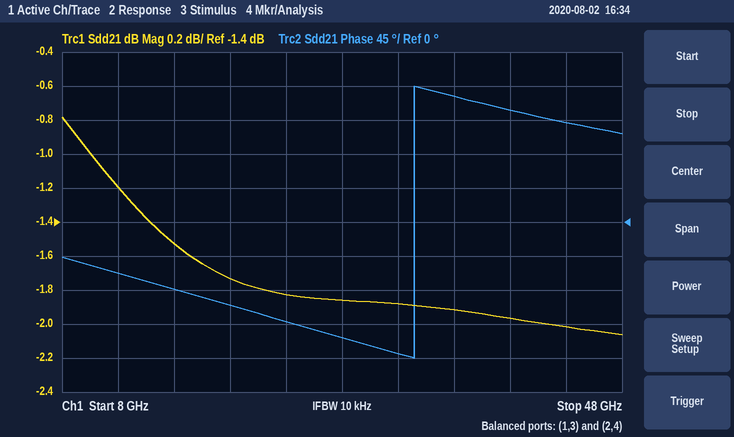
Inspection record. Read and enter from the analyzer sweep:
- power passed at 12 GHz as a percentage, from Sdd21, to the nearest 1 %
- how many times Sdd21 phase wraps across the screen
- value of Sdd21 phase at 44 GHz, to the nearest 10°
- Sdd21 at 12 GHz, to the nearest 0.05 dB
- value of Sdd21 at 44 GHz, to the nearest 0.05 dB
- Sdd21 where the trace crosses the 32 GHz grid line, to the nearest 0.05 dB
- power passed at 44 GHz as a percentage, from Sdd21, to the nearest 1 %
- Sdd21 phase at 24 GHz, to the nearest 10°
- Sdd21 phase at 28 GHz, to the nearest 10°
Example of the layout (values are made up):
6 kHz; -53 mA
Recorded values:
76 %; 1; 130°; -1.20 dB; -2.00 dB; -1.90 dB; 63 %; -130°; -150°
